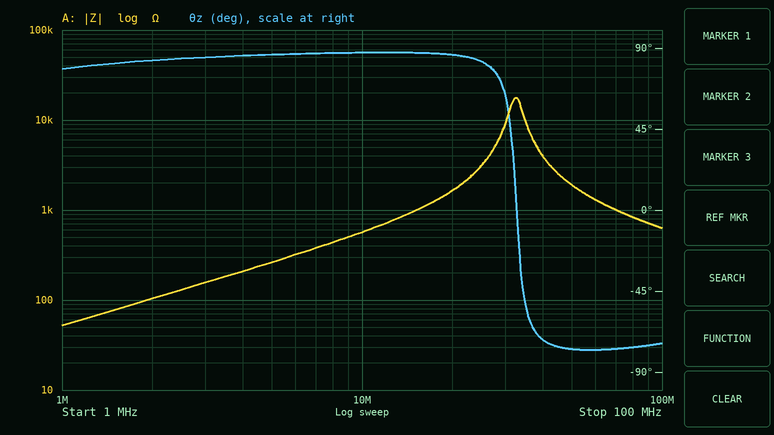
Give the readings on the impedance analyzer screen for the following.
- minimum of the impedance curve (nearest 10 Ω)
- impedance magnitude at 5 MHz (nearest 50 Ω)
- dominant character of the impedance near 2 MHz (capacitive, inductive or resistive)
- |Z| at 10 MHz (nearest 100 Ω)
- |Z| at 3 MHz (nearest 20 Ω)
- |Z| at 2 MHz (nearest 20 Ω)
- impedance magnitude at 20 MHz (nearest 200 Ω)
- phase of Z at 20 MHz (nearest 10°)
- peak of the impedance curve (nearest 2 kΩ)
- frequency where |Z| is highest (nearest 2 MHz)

50 Ω
250 Ω
inductive
600 Ω
160 Ω
100 Ω
1.6 kΩ
90°
18 kΩ
32 MHz
